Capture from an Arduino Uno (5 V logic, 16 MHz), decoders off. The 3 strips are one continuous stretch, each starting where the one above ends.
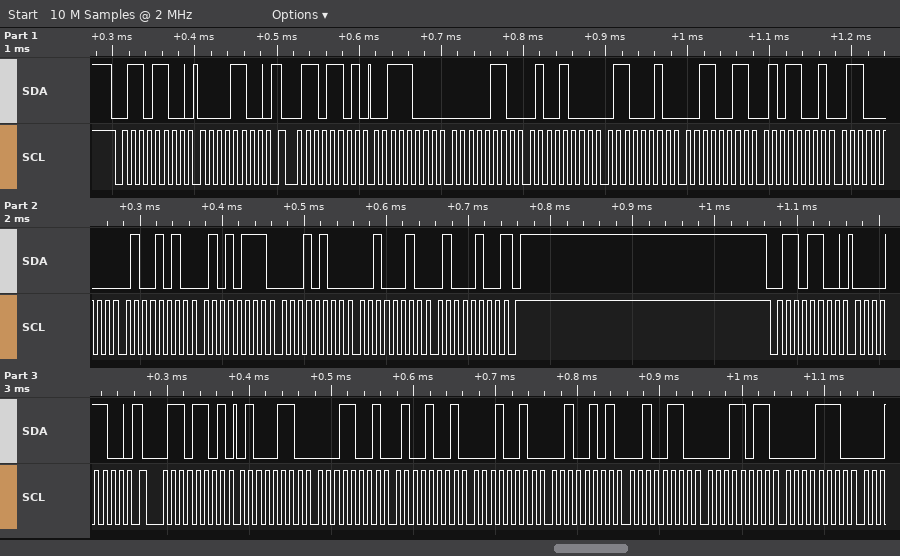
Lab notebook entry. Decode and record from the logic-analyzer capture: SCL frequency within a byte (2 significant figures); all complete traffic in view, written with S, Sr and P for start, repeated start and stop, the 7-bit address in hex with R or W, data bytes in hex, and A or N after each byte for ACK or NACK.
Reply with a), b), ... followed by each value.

a) 100 kHz
b) S 36W A 0C A Sr 36R A 38 A 06 A 48 A 62 A 33 A 59 A 60 A 4A A 57 A 14 A 22 A 44 N P S 36W A 0C A Sr 36R A 46 A 19 A 49 A 12 A 25 A 26 A 1B A 0E A
